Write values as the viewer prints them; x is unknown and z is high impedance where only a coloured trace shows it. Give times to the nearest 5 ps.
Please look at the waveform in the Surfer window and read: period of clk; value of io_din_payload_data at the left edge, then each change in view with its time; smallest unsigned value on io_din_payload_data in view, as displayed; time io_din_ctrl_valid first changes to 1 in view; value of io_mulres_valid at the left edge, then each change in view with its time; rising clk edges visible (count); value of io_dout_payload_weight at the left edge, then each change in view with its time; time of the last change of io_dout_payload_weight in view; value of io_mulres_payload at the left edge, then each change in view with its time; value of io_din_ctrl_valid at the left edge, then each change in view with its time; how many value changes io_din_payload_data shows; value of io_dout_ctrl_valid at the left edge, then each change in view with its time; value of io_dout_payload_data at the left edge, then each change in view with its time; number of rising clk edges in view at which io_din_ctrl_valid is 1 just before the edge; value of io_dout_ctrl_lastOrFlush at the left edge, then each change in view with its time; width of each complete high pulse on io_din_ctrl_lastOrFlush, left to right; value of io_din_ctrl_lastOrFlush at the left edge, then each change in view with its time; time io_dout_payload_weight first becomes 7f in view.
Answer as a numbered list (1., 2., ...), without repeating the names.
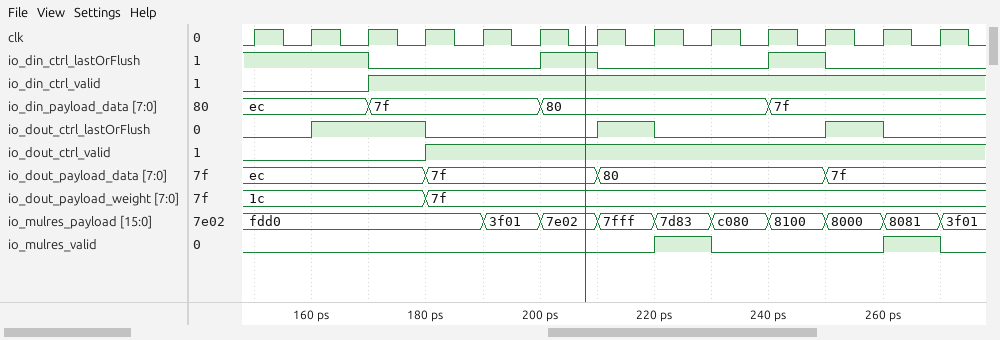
1. 10 ps
2. ec, 7f at 170 ps, 80 at 200 ps, 7f at 240 ps
3. 7f
4. 170 ps
5. 0, 1 at 220 ps, 0 at 230 ps, 1 at 260 ps, 0 at 270 ps
6. 13
7. 1c, 7f at 180 ps
8. 180 ps
9. fdd0, 3f01 at 190 ps, 7e02 at 200 ps, 7fff at 210 ps, 7d83 at 220 ps, c080 at 230 ps, 8100 at 240 ps, 8000 at 250 ps, 8081 at 260 ps, 3f01 at 270 ps
10. 0, 1 at 170 ps
11. 3
12. 0, 1 at 180 ps
13. ec, 7f at 180 ps, 80 at 210 ps, 7f at 250 ps
14. 10
15. 0, 1 at 160 ps, 0 at 180 ps, 1 at 210 ps, 0 at 220 ps, 1 at 250 ps, 0 at 260 ps
16. 10 ps, 10 ps
17. 1, 0 at 170 ps, 1 at 200 ps, 0 at 210 ps, 1 at 240 ps, 0 at 250 ps
18. 180 ps
